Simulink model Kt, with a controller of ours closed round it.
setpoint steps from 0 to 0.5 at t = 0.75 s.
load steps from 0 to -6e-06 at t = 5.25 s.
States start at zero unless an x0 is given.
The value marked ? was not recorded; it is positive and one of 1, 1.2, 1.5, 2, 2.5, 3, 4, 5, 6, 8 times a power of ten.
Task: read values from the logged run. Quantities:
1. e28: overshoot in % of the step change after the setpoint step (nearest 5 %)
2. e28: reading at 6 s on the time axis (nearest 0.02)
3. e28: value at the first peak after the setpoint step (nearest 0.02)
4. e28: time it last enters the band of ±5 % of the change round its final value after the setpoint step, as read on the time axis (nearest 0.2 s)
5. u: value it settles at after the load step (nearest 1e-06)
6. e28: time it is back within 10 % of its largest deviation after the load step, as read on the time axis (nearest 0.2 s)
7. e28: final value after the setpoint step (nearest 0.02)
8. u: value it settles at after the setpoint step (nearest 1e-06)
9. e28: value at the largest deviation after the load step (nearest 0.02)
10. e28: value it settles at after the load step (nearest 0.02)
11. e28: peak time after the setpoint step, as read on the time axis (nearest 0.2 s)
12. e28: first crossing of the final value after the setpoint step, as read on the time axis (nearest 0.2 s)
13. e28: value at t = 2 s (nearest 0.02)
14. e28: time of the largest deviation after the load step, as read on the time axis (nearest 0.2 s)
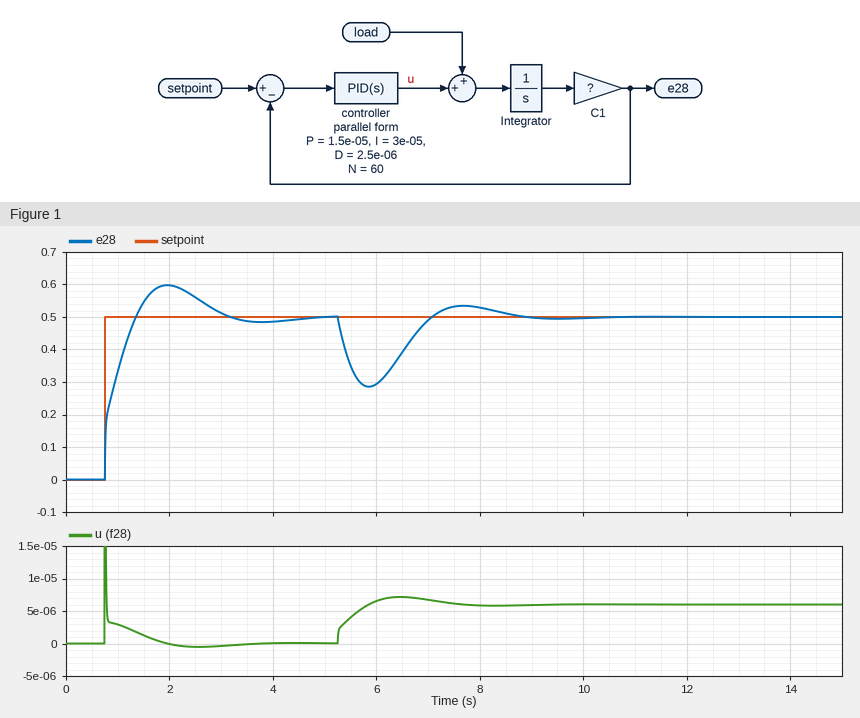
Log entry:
20 %
0.30
0.60
2.8 s
0.000006
8.2 s
0.50
0.000000
0.28
0.50
2.0 s
1.4 s
0.60
5.8 s
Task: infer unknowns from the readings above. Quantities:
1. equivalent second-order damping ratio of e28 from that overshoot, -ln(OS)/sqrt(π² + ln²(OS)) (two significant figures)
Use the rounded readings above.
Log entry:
0.46
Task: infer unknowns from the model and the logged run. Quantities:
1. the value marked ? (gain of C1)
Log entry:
200000
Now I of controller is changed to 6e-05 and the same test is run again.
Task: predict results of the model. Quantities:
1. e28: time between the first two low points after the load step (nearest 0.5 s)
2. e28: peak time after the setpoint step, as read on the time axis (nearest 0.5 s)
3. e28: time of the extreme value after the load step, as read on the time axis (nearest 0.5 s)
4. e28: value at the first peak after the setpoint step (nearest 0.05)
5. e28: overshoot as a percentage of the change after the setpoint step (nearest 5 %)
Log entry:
2.5 s
1.5 s
5.5 s
0.65
25 %
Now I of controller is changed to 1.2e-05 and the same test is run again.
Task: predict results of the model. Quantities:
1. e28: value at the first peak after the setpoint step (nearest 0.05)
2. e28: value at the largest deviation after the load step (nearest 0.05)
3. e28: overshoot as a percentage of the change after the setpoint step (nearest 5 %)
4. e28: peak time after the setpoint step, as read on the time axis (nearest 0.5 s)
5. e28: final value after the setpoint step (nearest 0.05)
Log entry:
0.55
0.25
10 %
2.5 s
0.50
